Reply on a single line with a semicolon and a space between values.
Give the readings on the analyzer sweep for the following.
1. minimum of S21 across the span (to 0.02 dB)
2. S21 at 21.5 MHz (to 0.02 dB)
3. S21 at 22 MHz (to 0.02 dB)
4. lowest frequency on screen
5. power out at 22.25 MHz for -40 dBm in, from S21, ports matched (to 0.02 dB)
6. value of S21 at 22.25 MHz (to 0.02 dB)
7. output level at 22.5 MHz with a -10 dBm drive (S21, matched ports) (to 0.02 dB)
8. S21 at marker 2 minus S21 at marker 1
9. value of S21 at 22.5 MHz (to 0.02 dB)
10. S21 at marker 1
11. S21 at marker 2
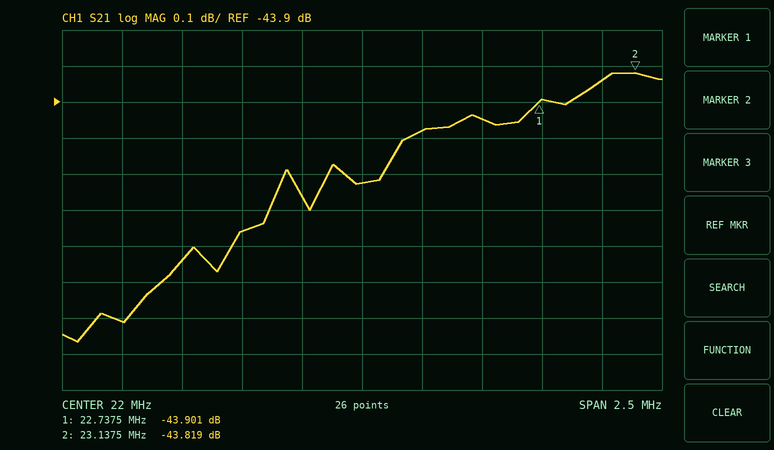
-44.56 dB; -44.26 dB; -44.12 dB; 20.75 MHz; -83.98 dBm; -43.98 dB; -53.94 dBm; 0.082 dB; -43.94 dB; -43.901 dB; -43.819 dB
